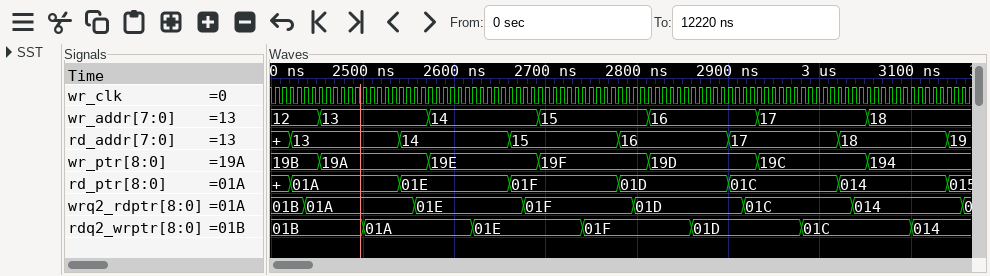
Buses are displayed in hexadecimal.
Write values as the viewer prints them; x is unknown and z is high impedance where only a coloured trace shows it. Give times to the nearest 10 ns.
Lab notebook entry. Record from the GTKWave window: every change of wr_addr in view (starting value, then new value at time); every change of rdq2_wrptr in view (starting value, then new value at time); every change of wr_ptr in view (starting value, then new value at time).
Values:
12, 13 at 2450 ns, 14 at 2570 ns, 15 at 2690 ns, 16 at 2810 ns, 17 at 2930 ns, 18 at 3050 ns
01B, 01A at 2500 ns, 01E at 2620 ns, 01F at 2740 ns, 01D at 2860 ns, 01C at 2980 ns, 014 at 3100 ns
19B, 19A at 2450 ns, 19E at 2570 ns, 19F at 2690 ns, 19D at 2810 ns, 19C at 2930 ns, 194 at 3050 ns
